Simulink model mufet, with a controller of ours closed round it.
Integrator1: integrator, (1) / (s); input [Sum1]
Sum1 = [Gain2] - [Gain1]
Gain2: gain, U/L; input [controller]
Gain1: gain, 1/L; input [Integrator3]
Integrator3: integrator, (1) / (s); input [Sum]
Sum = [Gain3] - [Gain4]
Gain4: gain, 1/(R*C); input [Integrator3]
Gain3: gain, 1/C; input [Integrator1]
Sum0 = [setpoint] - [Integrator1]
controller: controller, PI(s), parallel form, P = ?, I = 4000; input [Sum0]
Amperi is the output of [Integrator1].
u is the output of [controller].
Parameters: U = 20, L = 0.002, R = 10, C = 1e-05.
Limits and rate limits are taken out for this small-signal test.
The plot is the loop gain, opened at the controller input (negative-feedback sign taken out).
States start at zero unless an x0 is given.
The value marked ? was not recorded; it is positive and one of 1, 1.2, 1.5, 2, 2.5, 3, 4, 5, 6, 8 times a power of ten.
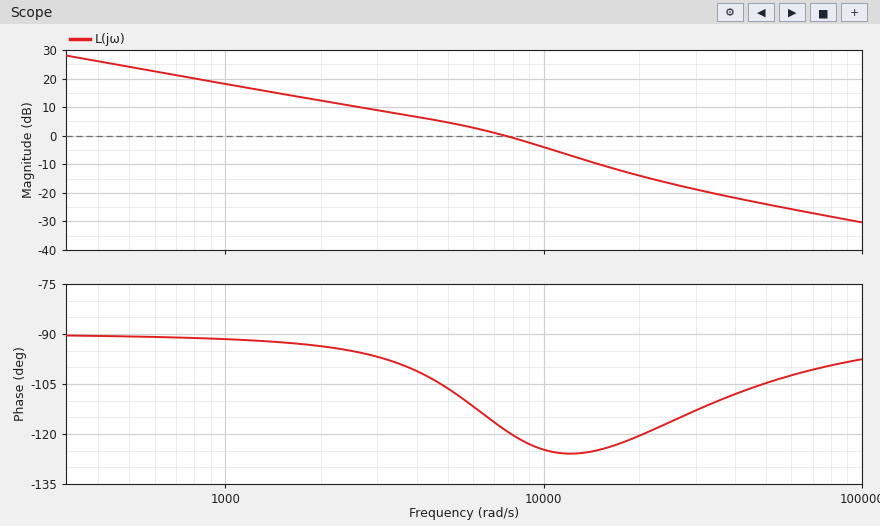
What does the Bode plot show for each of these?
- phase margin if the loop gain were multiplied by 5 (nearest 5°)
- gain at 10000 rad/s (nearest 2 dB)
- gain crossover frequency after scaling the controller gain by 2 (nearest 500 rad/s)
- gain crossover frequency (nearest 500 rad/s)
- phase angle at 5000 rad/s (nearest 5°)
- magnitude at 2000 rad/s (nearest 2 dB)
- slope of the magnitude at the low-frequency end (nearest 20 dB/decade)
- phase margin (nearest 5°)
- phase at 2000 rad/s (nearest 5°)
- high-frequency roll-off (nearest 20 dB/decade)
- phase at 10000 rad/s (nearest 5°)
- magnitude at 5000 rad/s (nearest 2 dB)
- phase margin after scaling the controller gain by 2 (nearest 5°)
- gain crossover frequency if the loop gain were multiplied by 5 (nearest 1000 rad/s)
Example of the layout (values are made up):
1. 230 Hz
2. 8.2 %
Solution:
1. 60°
2. -4 dB
3. 11500 rad/s
4. 7500 rad/s
5. -105°
6. 12 dB
7. -20 dB/decade
8. 60°
9. -95°
10. -20 dB/decade
11. -125°
12. 4 dB
13. 55°
14. 20000 rad/s
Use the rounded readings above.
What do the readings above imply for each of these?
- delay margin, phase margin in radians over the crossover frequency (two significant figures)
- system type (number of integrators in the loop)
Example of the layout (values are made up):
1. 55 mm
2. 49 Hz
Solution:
1. 0.00014 s
2. 1
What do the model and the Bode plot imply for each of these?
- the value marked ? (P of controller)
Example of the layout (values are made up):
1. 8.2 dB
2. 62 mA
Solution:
1. 0.3
